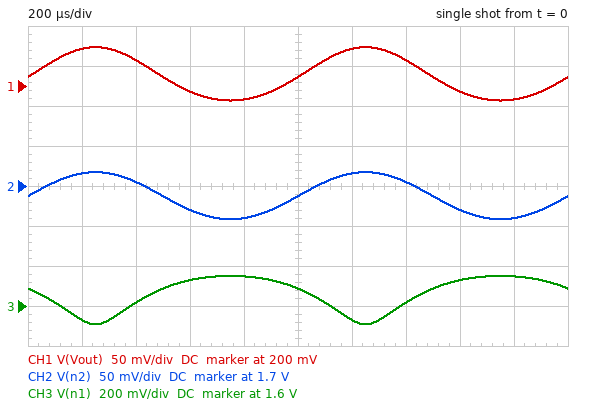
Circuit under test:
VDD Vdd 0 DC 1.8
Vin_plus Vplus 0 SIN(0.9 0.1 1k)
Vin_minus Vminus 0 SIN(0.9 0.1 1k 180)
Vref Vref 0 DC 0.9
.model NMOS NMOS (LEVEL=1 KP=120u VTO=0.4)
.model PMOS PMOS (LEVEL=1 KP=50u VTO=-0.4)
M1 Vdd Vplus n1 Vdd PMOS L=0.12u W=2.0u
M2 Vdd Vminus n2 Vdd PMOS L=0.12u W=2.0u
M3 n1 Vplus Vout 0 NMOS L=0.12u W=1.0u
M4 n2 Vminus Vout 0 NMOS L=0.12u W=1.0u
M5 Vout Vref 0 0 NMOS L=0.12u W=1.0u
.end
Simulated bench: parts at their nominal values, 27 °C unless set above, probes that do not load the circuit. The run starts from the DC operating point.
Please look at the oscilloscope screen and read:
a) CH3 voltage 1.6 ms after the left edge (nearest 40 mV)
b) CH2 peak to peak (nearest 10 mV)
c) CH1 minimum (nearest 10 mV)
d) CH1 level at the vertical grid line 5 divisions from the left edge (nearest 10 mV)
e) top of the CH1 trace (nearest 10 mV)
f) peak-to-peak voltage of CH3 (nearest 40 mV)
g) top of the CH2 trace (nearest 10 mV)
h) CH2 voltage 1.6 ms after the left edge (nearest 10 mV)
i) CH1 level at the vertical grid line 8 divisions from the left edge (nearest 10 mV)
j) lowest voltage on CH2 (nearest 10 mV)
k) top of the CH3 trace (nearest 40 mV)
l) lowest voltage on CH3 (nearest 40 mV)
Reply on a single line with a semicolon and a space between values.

1.72 V; 60 mV; 180 mV; 210 mV; 250 mV; 240 mV; 1.72 V; 1.67 V; 190 mV; 1.66 V; 1.76 V; 1.52 V
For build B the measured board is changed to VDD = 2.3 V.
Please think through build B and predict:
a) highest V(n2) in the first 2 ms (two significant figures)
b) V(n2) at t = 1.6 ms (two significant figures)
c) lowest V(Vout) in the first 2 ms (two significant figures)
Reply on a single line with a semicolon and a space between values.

2.3 V; 2.2 V; 180 mV
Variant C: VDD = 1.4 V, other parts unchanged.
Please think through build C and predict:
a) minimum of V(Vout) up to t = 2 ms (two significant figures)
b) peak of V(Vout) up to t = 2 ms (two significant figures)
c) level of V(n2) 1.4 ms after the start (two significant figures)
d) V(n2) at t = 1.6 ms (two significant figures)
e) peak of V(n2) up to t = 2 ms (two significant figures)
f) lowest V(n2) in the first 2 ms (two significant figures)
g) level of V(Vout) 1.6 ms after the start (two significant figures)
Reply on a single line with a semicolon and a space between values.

8.4 mV; 44 mV; 18 mV; 39 mV; 53 mV; 17 mV; 30 mV
